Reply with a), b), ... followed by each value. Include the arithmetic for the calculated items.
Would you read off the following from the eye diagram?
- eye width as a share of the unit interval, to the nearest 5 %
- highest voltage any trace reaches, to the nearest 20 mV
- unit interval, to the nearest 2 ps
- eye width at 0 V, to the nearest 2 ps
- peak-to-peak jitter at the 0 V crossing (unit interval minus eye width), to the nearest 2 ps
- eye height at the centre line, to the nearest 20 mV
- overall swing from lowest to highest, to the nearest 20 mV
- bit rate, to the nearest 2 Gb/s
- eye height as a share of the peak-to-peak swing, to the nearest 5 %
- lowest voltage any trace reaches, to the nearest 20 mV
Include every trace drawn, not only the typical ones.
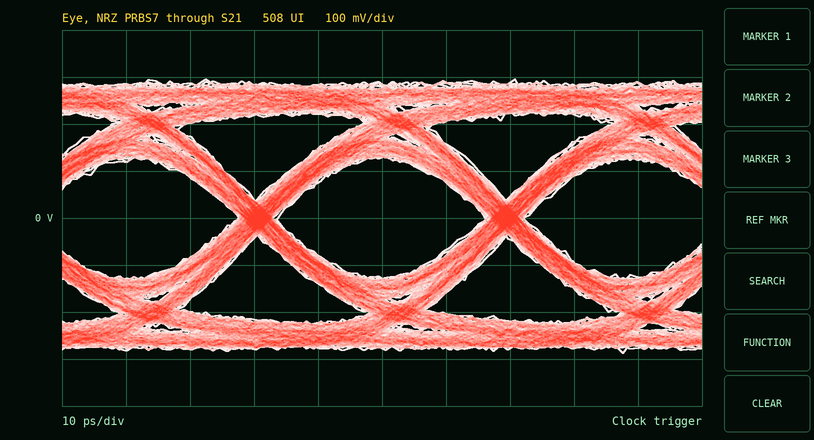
a) 32 ps / 38 ps ≈ 84.2 %, so 85 % to the nearest 5 %
b) 300 mV
c) 38 ps
d) 32 ps
e) 6 ps
f) 260 mV
g) 580 mV
h) 26 Gb/s
i) 260 mV / 580 mV ≈ 45 %
j) -280 mV
